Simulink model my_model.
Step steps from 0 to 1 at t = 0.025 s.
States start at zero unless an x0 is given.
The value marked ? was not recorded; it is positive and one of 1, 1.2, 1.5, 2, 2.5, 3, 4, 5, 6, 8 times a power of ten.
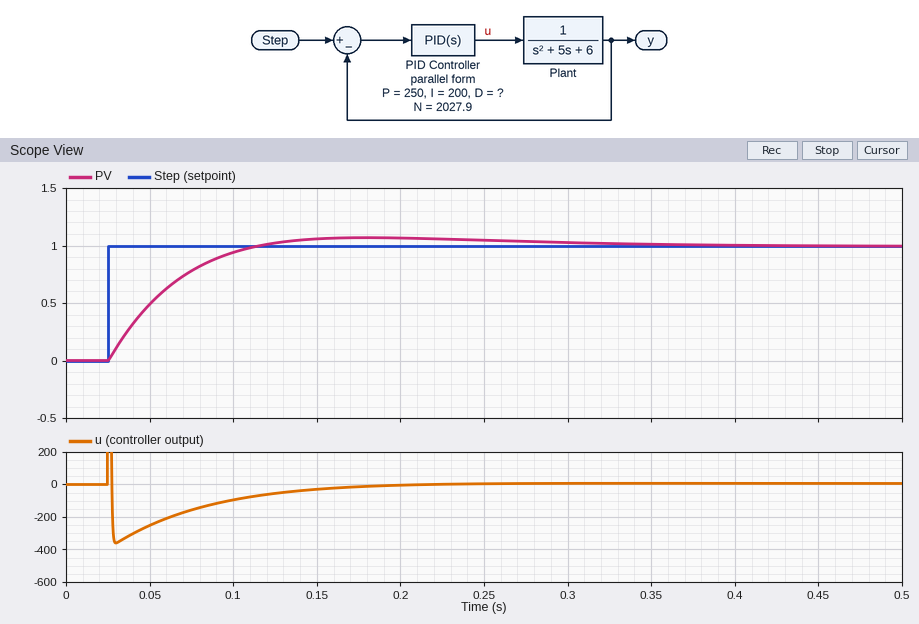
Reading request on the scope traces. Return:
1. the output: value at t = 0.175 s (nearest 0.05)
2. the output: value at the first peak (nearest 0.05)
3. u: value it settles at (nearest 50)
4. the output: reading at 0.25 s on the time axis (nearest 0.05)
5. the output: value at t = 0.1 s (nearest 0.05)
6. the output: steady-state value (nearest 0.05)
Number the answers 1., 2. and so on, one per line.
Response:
1. 1.05
2. 1.05
3. 0
4. 1.05
5. 0.95
6. 1.00
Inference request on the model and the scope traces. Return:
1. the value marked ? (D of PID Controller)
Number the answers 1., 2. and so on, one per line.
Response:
1. 25
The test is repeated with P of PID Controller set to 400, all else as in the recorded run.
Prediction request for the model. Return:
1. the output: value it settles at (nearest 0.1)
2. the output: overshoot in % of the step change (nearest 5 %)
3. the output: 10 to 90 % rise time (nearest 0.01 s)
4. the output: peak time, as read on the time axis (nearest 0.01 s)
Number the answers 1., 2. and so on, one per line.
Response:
1. 1.0
2. 15 %
3. 0.05 s
4. 0.15 s
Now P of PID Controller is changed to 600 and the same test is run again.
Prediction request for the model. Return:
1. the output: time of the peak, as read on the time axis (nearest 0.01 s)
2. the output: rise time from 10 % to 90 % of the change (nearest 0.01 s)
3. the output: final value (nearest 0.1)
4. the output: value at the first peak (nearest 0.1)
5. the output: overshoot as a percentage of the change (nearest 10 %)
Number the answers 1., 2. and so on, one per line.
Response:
1. 0.13 s
2. 0.04 s
3. 1.0
4. 1.2
5. 20 %
